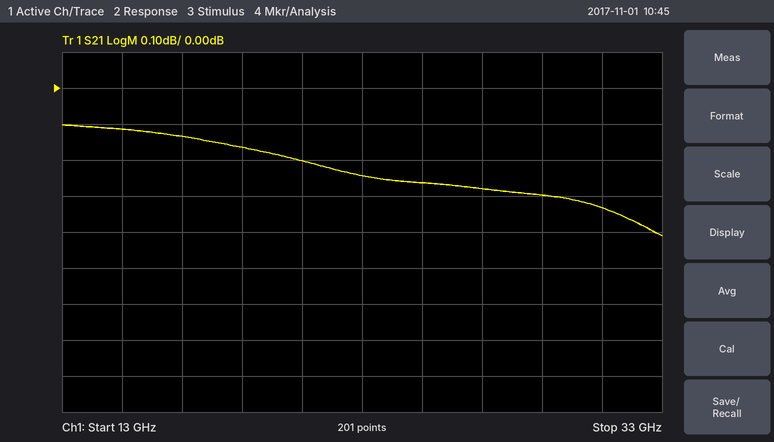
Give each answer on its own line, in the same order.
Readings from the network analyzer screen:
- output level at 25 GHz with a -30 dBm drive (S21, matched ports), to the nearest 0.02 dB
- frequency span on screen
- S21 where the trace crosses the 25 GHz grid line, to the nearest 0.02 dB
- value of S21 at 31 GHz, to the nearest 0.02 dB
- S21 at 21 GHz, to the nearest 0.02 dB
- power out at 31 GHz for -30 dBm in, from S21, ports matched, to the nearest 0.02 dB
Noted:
-30.26 dBm
20 GHz
-0.26 dB
-0.34 dB
-0.20 dB
-30.34 dBm
